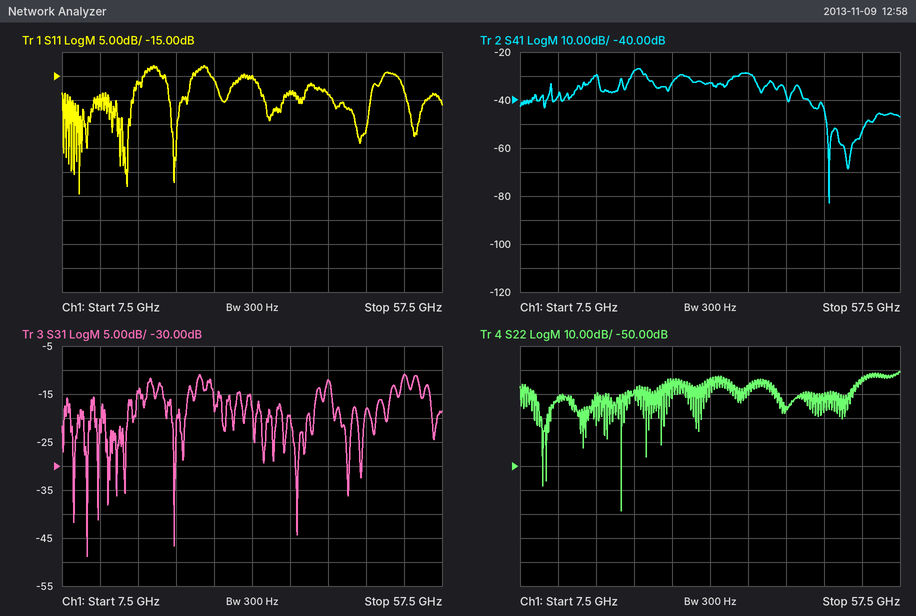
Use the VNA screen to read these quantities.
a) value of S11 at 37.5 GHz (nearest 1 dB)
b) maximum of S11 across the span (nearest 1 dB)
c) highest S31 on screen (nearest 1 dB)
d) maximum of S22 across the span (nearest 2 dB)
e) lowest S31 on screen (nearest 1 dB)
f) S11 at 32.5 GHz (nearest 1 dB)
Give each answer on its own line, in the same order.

-18 dB
-13 dB
-11 dB
-10 dB
-49 dB
-15 dB
